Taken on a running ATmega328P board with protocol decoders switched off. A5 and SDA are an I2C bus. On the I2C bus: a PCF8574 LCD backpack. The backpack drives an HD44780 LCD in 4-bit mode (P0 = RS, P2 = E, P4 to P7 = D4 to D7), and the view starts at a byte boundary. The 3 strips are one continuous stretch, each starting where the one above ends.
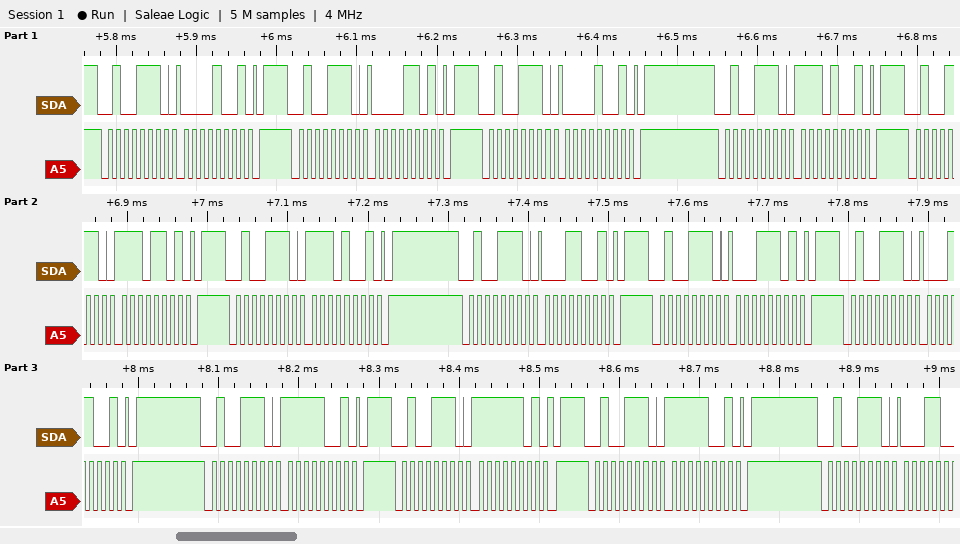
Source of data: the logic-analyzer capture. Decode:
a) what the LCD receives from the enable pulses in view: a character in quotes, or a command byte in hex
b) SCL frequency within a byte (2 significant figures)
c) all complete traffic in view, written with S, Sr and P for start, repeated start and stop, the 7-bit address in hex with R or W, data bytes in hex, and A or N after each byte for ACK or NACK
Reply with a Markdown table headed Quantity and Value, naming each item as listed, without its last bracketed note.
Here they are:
| Quantity | Value |
|---|---|
| what the LCD receives from the enable pulses in view: a character in quotes, or a command byte in hex | data 0x0E data 0x1F |
| SCL frequency within a byte | 100 kHz |
| all complete traffic in view, written with S, Sr and P for start, repeated start and stop, the 7-bit address in hex with R or W, data bytes in hex, and A or N after each byte for ACK or NACK | S 27W A 09 A P S 27W A 0D A P S 27W A 09 A P S 27W A E9 A P S 27W A ED A P S 27W A E9 A P S 27W A 19 A P S 27W A 1D A P S 27W A 19 A P S 27W A F9 A P S 27W A FD A P S 27W A F9 A P S 27W A |
